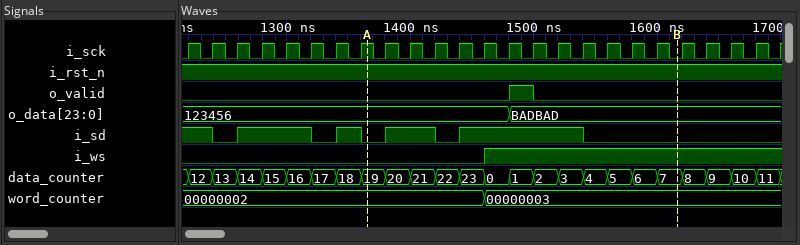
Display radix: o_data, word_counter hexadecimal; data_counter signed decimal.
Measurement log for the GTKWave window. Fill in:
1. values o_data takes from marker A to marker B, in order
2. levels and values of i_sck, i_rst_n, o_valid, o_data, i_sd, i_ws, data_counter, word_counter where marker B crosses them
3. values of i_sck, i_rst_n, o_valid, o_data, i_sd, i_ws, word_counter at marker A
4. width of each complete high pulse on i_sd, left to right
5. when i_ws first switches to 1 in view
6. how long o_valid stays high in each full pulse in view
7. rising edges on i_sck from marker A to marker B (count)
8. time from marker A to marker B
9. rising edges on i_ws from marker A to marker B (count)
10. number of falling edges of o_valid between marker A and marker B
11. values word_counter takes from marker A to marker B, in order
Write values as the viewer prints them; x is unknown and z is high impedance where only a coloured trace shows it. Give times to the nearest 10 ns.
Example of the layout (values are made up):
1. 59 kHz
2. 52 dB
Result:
1. 123456, BADBAD
2. i_sck=0, i_rst_n=1, o_valid=0, o_data=BADBAD, i_sd=0, i_ws=1, data_counter=7, word_counter=00000003
3. i_sck=1, i_rst_n=1, o_valid=0, o_data=123456, i_sd=0, i_ws=0, word_counter=00000002
4. 60 ns, 20 ns, 40 ns, 100 ns
5. 1460 ns
6. 20 ns
7. 12
8. 250 ns
9. 1
10. 1
11. 00000002, 00000003
